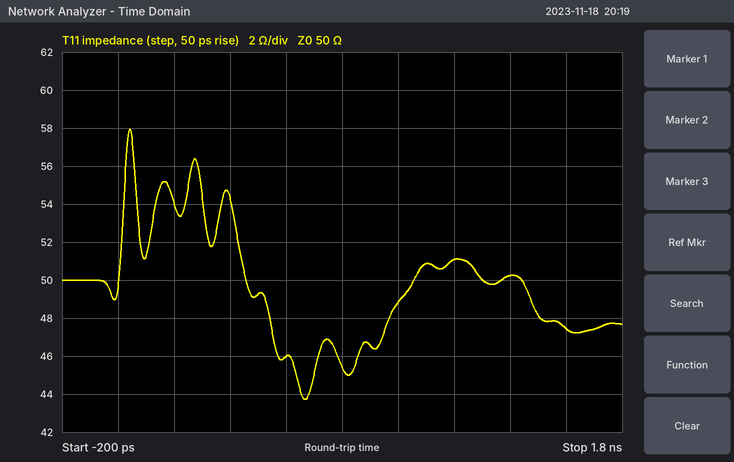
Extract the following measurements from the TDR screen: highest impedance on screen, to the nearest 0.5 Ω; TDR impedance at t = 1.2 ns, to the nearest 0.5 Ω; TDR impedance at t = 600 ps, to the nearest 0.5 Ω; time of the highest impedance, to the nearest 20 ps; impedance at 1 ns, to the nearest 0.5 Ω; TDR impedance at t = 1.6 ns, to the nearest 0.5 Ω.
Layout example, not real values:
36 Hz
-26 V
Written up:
58.0 Ω
51.0 Ω
46.0 Ω
40 ps
49.0 Ω
47.5 Ω
